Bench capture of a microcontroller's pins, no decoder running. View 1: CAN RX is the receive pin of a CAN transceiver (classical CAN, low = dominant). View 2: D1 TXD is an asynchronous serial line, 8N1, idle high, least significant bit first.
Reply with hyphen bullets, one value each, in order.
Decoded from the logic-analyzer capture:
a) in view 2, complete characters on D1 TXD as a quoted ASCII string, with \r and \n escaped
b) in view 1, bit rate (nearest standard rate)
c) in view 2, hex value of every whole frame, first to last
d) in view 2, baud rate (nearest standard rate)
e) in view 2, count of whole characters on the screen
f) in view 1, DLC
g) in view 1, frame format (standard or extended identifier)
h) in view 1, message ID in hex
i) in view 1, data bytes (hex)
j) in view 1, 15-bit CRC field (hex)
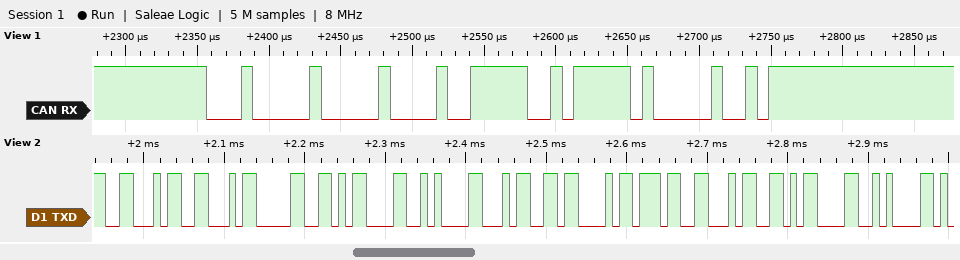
- "FF0\r\n4C74\r\n"
- 125 kbit/s
- 46 46 30 0D 0A 34 43 37 34 0D 0A
- 115200 baud
- 11
- 1
- standard
- 0x100
- 3E
- 0x5F80
